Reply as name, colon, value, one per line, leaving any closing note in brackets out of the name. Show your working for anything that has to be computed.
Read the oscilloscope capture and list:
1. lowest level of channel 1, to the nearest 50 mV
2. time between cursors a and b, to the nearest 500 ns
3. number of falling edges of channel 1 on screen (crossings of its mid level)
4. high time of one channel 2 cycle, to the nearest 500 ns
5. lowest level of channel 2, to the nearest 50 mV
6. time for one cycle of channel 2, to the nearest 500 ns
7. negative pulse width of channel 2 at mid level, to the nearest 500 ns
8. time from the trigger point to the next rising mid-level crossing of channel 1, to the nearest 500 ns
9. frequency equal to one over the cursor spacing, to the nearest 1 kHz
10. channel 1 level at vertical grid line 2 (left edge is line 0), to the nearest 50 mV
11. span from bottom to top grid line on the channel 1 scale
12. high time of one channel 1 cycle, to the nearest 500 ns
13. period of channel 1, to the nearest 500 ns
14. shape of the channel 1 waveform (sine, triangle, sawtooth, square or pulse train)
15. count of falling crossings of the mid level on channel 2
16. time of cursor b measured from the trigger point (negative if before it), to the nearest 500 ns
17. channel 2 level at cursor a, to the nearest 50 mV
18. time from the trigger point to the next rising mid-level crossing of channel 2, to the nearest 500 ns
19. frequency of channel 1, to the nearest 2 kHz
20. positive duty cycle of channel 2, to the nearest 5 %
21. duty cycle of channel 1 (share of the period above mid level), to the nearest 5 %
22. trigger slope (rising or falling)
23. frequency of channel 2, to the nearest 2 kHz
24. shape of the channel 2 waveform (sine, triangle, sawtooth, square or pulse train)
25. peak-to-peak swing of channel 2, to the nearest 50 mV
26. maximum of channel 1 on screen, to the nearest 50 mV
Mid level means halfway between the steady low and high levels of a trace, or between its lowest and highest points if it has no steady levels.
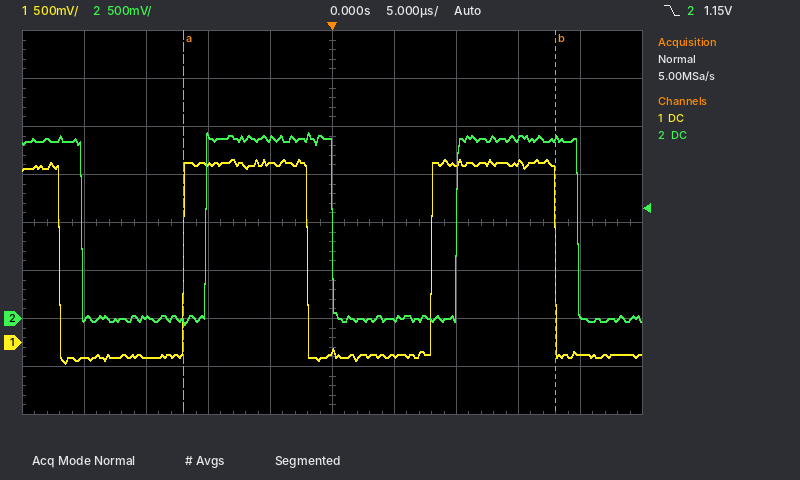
lowest level of channel 1, to the nearest 50 mV: -200 mV
time between cursors a and b, to the nearest 500 ns: 30.0 µs
number of falling edges of channel 1 on screen: 3
high time of one channel 2 cycle, to the nearest 500 ns: 10.0 µs
lowest level of channel 2, to the nearest 50 mV: -50 mV
time for one cycle of channel 2, to the nearest 500 ns: 20.0 µs
negative pulse width of channel 2 at mid level, to the nearest 500 ns: 10.0 µs
time from the trigger point to the next rising mid-level crossing of channel 1, to the nearest 500 ns: 8.0 µs
frequency equal to one over the cursor spacing, to the nearest 1 kHz: 1 / 30.0 µs ≈ 33 kHz
channel 1 level at vertical grid line 2 (left edge is line 0), to the nearest 50 mV: -150 mV
span from bottom to top grid line on the channel 1 scale: 4 V
high time of one channel 1 cycle, to the nearest 500 ns: 10.0 µs
period of channel 1, to the nearest 500 ns: 20.0 µs
shape of the channel 1 waveform: square
count of falling crossings of the mid level on channel 2: 3
time of cursor b measured from the trigger point (negative if before it), to the nearest 500 ns: +18.0 µs
channel 2 level at cursor a, to the nearest 50 mV: -50 mV
time from the trigger point to the next rising mid-level crossing of channel 2, to the nearest 500 ns: 10.0 µs
frequency of channel 1, to the nearest 2 kHz: 1 / 20.0 µs ≈ 50 kHz
positive duty cycle of channel 2, to the nearest 5 %: 10.0 µs / 20.0 µs ≈ 50 %
duty cycle of channel 1 (share of the period above mid level), to the nearest 5 %: 10.0 µs / 20.0 µs ≈ 50 %
trigger slope: falling
frequency of channel 2, to the nearest 2 kHz: 1 / 20.0 µs ≈ 50 kHz
shape of the channel 2 waveform: square
peak-to-peak swing of channel 2, to the nearest 50 mV: 1.95 V − (-50 mV) = 2.00 V
maximum of channel 1 on screen, to the nearest 50 mV: 1.90 V
